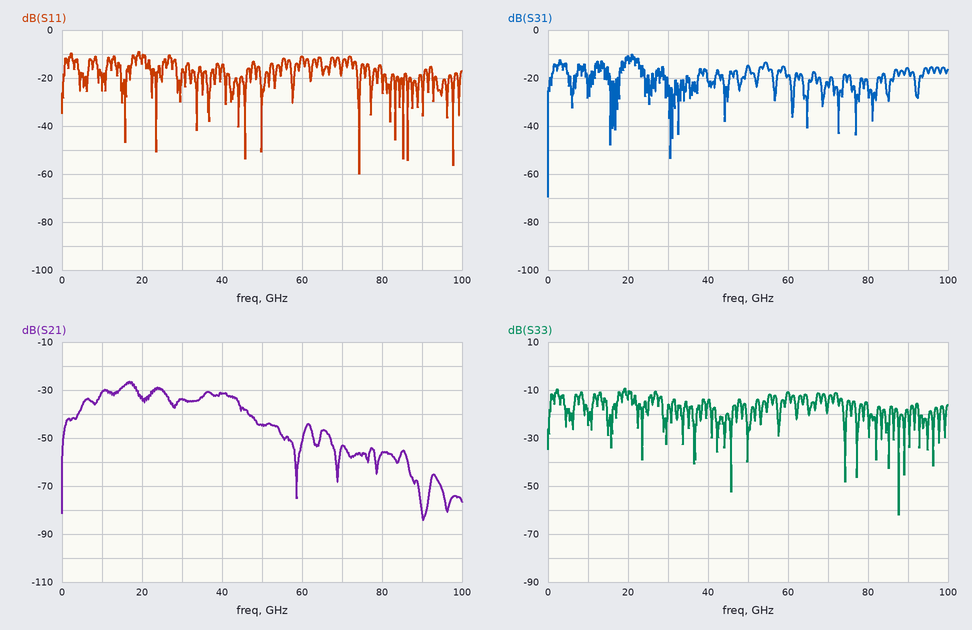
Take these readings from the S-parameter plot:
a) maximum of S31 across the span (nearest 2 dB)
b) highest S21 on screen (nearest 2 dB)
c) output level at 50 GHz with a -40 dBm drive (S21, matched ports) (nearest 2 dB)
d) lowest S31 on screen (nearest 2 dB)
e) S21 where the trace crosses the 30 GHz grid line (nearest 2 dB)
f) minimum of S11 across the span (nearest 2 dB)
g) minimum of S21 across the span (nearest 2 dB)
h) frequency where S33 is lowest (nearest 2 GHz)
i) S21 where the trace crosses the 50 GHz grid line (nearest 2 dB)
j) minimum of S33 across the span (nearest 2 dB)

-10 dB
-26 dB
-84 dBm
-70 dB
-34 dB
-60 dB
-84 dB
88 GHz
-44 dB
-62 dB
